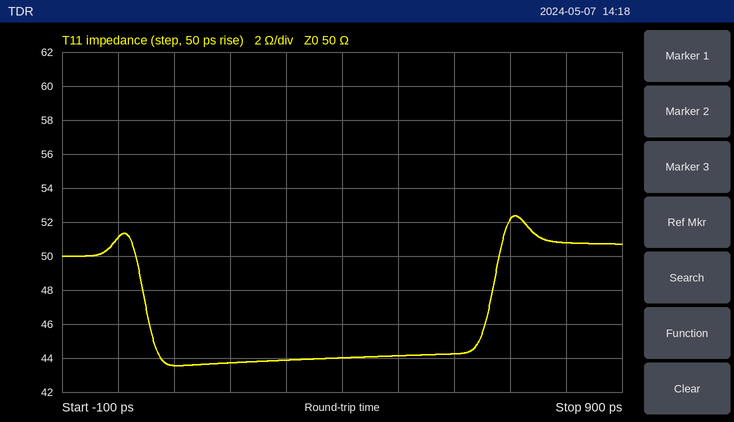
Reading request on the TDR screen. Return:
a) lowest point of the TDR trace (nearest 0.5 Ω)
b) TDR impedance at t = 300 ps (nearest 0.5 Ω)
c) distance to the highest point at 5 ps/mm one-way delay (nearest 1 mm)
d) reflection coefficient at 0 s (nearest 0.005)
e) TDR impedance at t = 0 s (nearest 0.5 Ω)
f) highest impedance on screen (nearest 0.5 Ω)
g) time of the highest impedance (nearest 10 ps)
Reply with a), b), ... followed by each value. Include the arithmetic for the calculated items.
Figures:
a) 43.5 Ω
b) 44.0 Ω
c) 710 ps / 2 / 5 ps/mm ≈ 71 mm
d) (51 − 50)/(51 + 50) ≈ +0.010
e) 51.0 Ω
f) 52.5 Ω
g) 710 ps
